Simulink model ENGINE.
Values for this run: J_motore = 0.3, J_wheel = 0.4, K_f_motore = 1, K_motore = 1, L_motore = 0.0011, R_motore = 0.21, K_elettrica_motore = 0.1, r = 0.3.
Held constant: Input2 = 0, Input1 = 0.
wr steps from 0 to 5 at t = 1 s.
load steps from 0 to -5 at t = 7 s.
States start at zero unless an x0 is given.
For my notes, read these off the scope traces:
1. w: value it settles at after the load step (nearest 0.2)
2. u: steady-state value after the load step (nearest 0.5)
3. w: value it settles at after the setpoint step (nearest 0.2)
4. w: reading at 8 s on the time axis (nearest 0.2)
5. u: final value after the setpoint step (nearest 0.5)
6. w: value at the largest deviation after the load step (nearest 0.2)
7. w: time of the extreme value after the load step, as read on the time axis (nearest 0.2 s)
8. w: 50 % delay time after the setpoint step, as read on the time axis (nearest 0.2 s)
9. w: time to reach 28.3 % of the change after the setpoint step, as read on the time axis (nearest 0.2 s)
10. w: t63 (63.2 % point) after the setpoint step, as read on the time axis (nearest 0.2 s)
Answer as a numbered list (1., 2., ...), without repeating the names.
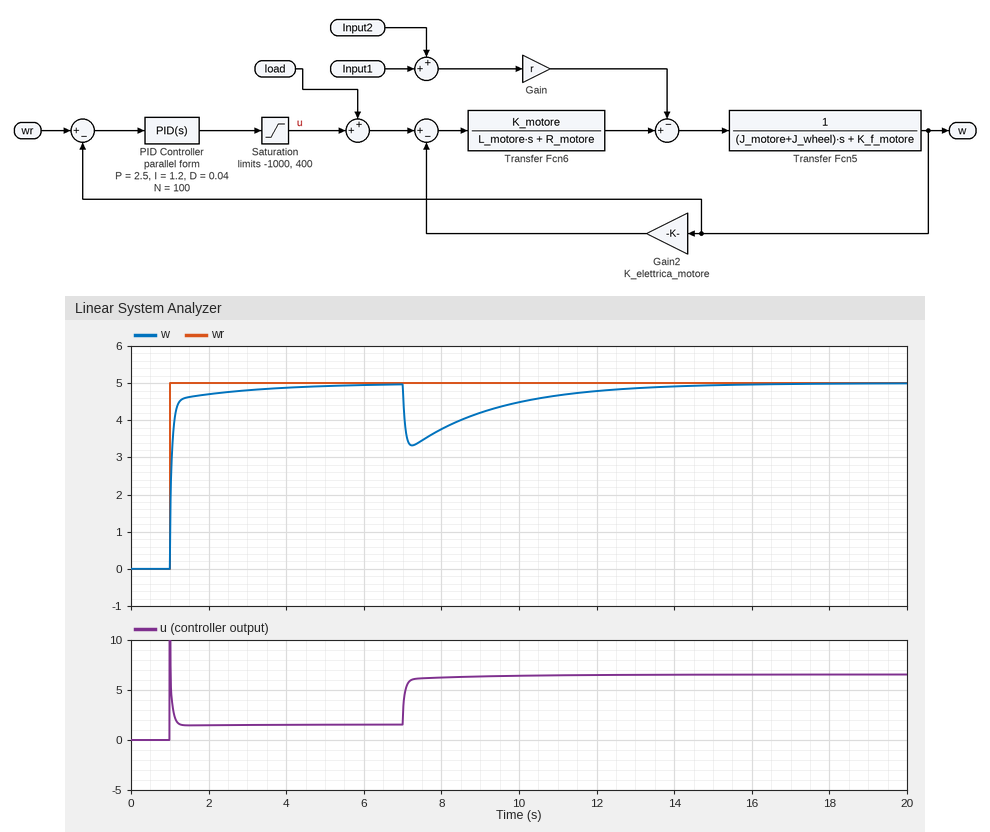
1. 5.0
2. 6.5
3. 5.0
4. 3.8
5. 1.5
6. 3.4
7. 7.2 s
8. 1.0 s
9. 1.0 s
10. 1.0 s
